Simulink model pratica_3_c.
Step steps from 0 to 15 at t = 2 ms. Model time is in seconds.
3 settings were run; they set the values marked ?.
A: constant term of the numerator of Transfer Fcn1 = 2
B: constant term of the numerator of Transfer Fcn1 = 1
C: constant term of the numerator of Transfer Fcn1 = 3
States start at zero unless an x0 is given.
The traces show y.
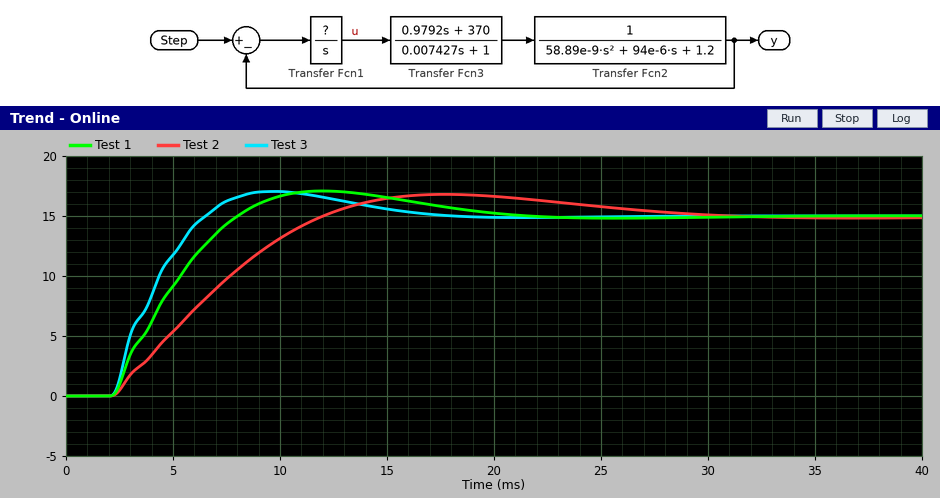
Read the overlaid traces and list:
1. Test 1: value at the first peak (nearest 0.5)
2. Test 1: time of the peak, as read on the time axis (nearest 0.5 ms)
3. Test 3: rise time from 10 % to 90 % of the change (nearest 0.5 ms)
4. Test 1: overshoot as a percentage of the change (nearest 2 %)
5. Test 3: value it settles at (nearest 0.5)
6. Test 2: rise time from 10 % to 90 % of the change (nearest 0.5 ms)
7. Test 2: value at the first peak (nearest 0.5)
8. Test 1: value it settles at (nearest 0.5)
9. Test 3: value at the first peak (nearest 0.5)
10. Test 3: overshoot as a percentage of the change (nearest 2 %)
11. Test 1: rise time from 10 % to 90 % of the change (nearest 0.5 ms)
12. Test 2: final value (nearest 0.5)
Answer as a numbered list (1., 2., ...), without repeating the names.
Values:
1. 17.0
2. 12.0 ms
3. 3.0 ms
4. 14 %
5. 15.0
6. 7.5 ms
7. 17.0
8. 15.0
9. 17.0
10. 14 %
11. 4.5 ms
12. 15.0
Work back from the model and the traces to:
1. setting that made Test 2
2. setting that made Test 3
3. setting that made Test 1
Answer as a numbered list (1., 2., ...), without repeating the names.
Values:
1. B
2. C
3. A
